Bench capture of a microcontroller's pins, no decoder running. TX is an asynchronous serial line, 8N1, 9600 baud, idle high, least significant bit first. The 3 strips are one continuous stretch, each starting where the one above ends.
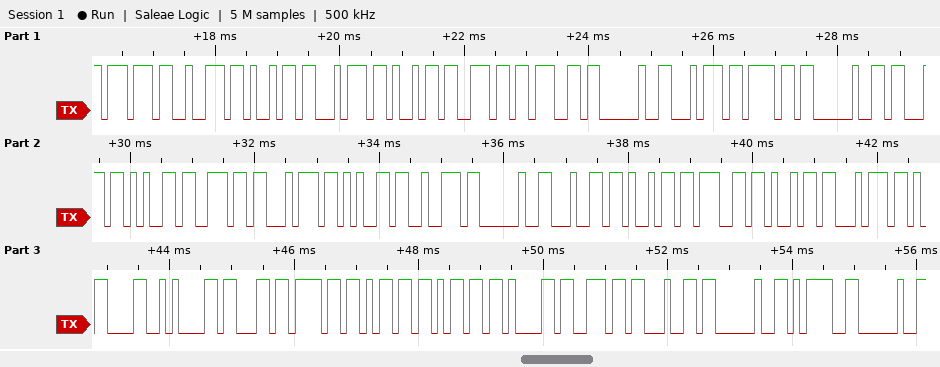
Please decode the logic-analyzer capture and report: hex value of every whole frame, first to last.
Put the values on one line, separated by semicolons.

77 72 69 74 69 6E 67 20 74 6F 20 63 65 6E 74 65 72 20 64 69 67 69 74 0D 0A 63 6F 6D 6D 61 6E 64 20 3D 20
